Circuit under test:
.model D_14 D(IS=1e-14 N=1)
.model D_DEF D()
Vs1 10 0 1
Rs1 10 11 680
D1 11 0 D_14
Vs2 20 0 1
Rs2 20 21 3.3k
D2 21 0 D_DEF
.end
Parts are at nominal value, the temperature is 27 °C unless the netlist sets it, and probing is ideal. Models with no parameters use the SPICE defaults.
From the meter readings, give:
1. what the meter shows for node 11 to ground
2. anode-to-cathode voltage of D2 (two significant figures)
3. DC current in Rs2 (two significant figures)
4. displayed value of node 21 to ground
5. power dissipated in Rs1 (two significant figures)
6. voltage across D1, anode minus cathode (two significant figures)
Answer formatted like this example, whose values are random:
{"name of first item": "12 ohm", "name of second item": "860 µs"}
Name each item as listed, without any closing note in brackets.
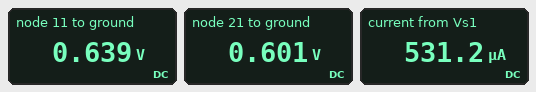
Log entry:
{"what the meter shows for node 11 to ground": "0.639 V", "anode-to-cathode voltage of D2": "600 mV", "DC current in Rs2": "120 µA", "displayed value of node 21 to ground": "0.601 V", "power dissipated in Rs1": "190 µW", "voltage across D1, anode minus cathode": "640 mV"}
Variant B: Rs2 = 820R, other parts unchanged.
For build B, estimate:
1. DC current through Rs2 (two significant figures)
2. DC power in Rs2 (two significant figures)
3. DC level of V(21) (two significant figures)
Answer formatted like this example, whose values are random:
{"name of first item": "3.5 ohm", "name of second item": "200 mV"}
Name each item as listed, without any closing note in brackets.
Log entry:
{"DC current through Rs2": "450 µA", "DC power in Rs2": "160 µW", "DC level of V(21)": "630 mV"}
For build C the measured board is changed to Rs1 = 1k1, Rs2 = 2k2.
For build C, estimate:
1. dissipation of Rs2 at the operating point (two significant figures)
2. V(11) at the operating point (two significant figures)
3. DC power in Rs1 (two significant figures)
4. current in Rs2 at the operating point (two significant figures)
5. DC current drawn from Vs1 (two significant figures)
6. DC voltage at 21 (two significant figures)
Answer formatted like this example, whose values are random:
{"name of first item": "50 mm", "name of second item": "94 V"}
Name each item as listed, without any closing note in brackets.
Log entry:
{"dissipation of Rs2 at the operating point": "69 µW", "V(11) at the operating point": "630 mV", "DC power in Rs1": "130 µW", "current in Rs2 at the operating point": "180 µA", "DC current drawn from Vs1": "340 µA", "DC voltage at 21": "610 mV"}
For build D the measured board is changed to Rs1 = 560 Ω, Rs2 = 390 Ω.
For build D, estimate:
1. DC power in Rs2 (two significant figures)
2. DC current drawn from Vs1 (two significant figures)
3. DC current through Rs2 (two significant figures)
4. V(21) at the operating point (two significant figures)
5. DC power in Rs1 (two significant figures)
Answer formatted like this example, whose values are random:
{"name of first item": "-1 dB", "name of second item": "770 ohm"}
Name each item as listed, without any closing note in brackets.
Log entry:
{"DC power in Rs2": "310 µW", "DC current drawn from Vs1": "640 µA", "DC current through Rs2": "890 µA", "V(21) at the operating point": "650 mV", "DC power in Rs1": "230 µW"}
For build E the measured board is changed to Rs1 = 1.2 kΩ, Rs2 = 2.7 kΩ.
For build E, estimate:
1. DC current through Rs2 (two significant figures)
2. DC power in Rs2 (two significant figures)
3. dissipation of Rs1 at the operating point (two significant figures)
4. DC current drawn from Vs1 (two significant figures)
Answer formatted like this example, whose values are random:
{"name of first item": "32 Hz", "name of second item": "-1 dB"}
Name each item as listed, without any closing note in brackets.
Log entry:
{"DC current through Rs2": "150 µA", "DC power in Rs2": "58 µW", "dissipation of Rs1 at the operating point": "120 µW", "DC current drawn from Vs1": "310 µA"}
